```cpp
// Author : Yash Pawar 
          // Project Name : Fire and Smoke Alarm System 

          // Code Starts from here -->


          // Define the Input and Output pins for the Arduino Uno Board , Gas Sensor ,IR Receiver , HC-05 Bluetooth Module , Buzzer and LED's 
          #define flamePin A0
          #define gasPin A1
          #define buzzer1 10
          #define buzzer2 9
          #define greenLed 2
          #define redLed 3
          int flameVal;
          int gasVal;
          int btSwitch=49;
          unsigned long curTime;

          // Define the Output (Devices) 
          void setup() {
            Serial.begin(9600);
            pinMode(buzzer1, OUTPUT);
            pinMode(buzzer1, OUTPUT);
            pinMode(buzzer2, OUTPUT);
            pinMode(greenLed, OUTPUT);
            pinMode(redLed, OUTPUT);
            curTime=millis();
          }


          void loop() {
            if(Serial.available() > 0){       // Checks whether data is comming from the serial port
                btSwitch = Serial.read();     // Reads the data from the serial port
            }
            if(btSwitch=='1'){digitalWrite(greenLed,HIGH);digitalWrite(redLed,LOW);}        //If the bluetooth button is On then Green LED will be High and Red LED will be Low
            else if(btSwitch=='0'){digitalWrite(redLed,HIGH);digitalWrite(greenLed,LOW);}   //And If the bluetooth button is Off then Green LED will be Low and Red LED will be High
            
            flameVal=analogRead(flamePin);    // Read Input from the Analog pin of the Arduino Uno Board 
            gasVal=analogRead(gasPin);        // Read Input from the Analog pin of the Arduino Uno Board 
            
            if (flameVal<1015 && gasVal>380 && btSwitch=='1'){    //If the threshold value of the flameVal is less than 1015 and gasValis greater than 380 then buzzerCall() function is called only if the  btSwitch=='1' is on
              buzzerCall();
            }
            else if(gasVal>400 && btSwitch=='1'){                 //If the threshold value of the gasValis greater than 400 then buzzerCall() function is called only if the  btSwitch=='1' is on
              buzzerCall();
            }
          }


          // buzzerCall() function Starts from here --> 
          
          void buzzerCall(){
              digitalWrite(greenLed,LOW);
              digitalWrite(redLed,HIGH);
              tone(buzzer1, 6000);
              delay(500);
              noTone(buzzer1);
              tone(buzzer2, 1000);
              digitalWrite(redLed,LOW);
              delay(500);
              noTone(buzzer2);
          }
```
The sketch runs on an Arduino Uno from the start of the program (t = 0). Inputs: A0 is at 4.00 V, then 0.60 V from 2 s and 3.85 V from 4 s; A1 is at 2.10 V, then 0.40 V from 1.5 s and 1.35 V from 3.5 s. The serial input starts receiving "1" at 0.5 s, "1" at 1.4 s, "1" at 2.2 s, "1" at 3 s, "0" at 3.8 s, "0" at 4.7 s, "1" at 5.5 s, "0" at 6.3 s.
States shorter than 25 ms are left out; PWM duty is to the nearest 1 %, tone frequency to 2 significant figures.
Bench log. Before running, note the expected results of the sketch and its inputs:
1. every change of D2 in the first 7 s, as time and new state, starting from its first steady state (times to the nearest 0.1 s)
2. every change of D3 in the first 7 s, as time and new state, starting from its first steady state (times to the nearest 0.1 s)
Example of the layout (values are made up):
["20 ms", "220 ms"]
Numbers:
["0 s low; 2 s high; 3.8 s low; 5.5 s high; 6.3 s low", "0 s high; 0.5 s low; 1 s high; 1.5 s low; 3.8 s high; 5.5 s low; 6.3 s high"]
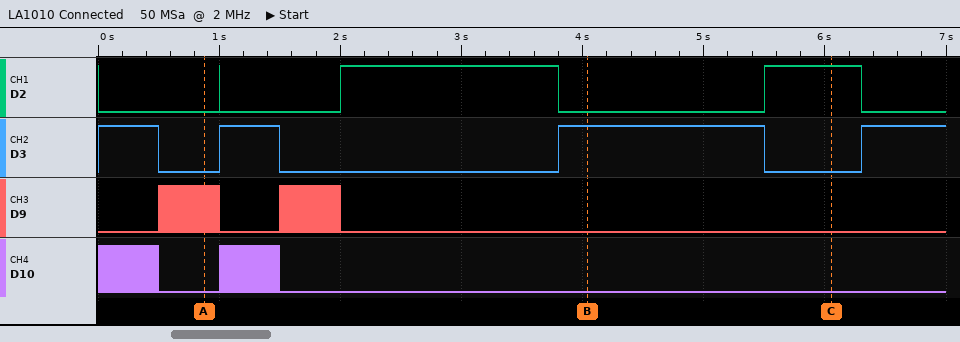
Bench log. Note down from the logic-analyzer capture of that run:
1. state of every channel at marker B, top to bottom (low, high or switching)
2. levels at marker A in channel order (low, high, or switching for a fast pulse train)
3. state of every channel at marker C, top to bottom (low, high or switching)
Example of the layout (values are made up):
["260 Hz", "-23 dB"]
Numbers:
["D2 low, D3 high, D9 low, D10 low", "D2 low, D3 low, D9 switching, D10 low", "D2 high, D3 low, D9 low, D10 low"]
